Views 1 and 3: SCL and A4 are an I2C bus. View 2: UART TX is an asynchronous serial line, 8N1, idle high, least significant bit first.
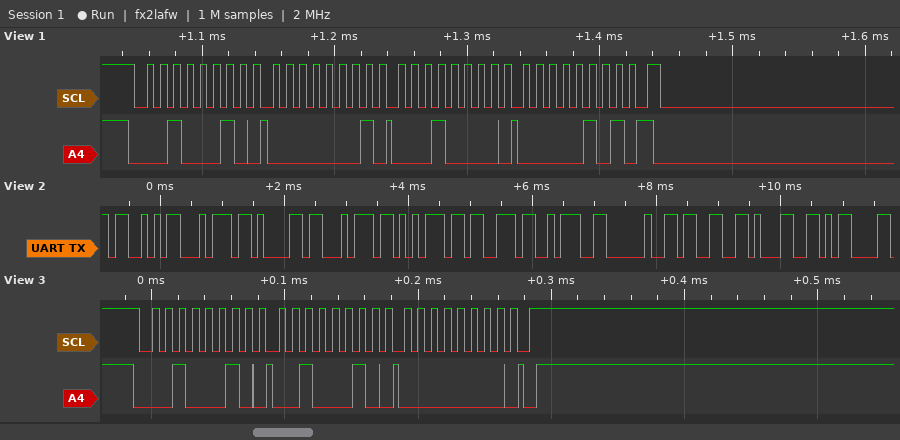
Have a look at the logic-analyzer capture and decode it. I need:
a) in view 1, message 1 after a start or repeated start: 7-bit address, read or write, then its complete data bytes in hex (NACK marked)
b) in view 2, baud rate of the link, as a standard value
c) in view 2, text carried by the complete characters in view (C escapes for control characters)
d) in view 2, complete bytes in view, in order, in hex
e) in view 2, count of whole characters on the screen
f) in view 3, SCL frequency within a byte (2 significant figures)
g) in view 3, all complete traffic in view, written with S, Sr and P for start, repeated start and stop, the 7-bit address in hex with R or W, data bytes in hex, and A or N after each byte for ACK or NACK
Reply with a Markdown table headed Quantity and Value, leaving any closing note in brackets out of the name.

| Quantity | Value |
|---|---|
| in view 1, message 1 after a start or repeated start: 7-bit address, read or write, then its complete data bytes in hex | 0x11 write: 01 10 05 |
| in view 2, baud rate of the link, as a standard value | 9600 baud |
| in view 2, text carried by the complete characters in view | "Status: 31\r" |
| in view 2, complete bytes in view, in order, in hex | 53 74 61 74 75 73 3A 20 33 31 0D |
| in view 2, count of whole characters on the screen | 11 |
| in view 3, SCL frequency within a byte | 100 kHz |
| in view 3, all complete traffic in view, written with S, Sr and P for start, repeated start and stop, the 7-bit address in hex with R or W, data bytes in hex, and A or N after each byte for ACK or NACK | S 11W A 22 A 00 A P |
